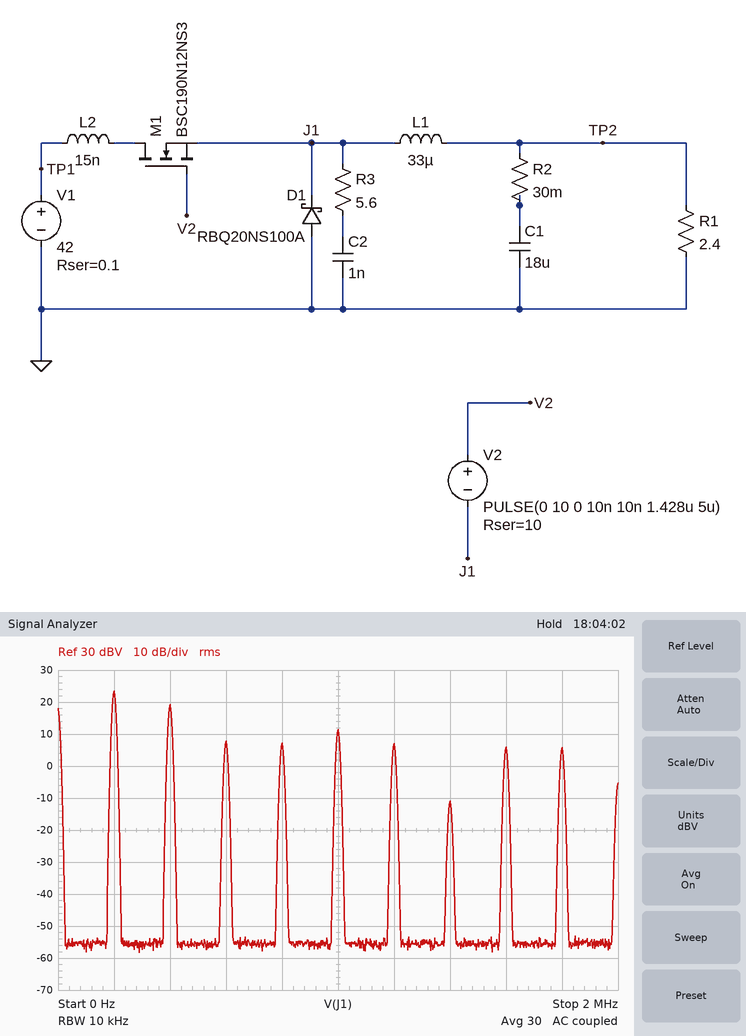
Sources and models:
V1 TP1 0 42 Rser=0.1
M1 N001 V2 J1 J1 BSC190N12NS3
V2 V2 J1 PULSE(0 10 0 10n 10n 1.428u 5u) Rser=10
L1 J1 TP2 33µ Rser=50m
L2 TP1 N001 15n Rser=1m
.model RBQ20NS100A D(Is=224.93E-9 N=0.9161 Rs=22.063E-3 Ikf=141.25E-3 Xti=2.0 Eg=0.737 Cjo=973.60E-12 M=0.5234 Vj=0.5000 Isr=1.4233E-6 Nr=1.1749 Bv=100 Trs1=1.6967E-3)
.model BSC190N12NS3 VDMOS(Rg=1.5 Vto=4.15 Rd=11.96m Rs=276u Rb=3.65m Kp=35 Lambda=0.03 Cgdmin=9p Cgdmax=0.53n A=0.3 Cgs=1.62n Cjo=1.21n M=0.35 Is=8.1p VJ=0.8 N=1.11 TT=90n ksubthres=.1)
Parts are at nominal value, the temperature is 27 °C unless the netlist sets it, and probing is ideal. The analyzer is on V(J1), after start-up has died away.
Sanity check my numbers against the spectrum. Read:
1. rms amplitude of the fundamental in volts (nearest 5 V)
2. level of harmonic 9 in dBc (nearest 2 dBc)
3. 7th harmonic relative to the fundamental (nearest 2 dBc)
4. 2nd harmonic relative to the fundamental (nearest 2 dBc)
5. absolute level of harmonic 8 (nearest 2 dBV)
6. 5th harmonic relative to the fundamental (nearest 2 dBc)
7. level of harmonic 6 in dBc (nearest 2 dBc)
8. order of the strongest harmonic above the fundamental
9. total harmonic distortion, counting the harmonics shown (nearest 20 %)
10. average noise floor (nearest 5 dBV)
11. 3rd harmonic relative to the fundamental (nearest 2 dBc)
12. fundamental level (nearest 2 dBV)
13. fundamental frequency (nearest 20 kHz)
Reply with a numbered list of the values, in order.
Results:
1. 15 V
2. -18 dBc
3. -34 dBc
4. -4 dBc
5. 6 dBV
6. -12 dBc
7. -16 dBc
8. 2
9. 80 %
10. -55 dBV
11. -16 dBc
12. 24 dBV
13. 200 kHz
